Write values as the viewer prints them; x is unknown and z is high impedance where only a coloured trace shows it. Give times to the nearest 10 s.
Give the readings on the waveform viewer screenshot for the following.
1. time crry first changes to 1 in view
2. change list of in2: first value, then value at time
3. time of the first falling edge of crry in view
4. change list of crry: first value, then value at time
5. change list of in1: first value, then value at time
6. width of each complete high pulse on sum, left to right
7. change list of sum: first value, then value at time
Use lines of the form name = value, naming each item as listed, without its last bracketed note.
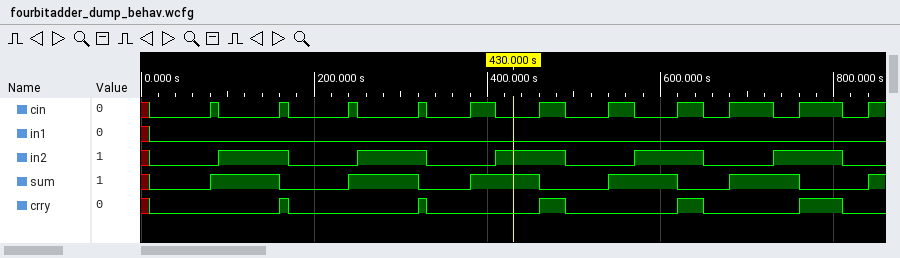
time crry first changes to 1 in view = 160 s
change list of in2: first value, then value at time = x, 0 at 10 s, 1 at 90 s, 0 at 170 s, 1 at 250 s, 0 at 330 s, 1 at 410 s, 0 at 490 s, 1 at 570 s, 0 at 650 s, 1 at 730 s, 0 at 810 s
time of the first falling edge of crry in view = 170 s
change list of crry: first value, then value at time = x, 0 at 10 s, 1 at 160 s, 0 at 170 s, 1 at 320 s, 0 at 330 s, 1 at 460 s, 0 at 490 s, 1 at 620 s, 0 at 650 s, 1 at 760 s, 0 at 810 s
change list of in1: first value, then value at time = x, 0 at 10 s
width of each complete high pulse on sum, left to right = 80 s, 80 s, 80 s, 80 s, 80 s
change list of sum: first value, then value at time = x, 0 at 10 s, 1 at 80 s, 0 at 160 s, 1 at 240 s, 0 at 320 s, 1 at 380 s, 0 at 460 s, 1 at 540 s, 0 at 620 s, 1 at 680 s, 0 at 760 s, 1 at 840 s
